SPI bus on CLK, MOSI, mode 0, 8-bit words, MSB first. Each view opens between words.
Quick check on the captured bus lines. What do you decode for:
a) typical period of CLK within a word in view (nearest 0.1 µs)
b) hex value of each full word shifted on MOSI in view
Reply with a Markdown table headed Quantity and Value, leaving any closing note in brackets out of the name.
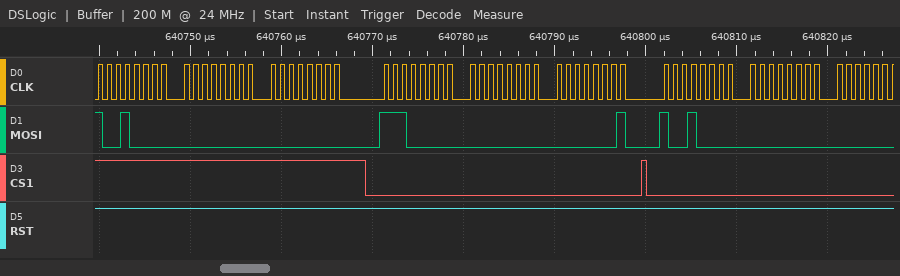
| Quantity | Value |
|---|---|
| typical period of CLK within a word in view | 1 µs |
| hex value of each full word shifted on MOSI in view | 90, 00, 00, E0, 00, 01, 90, 00 |
